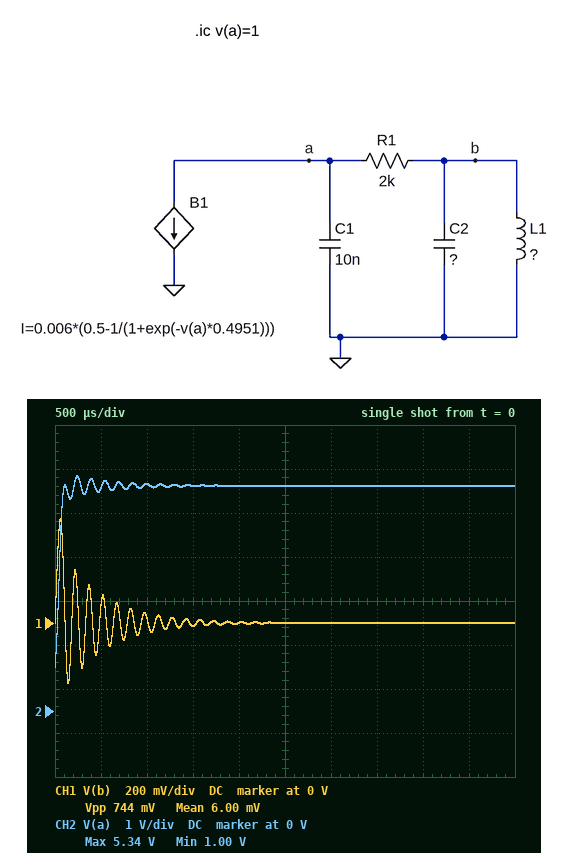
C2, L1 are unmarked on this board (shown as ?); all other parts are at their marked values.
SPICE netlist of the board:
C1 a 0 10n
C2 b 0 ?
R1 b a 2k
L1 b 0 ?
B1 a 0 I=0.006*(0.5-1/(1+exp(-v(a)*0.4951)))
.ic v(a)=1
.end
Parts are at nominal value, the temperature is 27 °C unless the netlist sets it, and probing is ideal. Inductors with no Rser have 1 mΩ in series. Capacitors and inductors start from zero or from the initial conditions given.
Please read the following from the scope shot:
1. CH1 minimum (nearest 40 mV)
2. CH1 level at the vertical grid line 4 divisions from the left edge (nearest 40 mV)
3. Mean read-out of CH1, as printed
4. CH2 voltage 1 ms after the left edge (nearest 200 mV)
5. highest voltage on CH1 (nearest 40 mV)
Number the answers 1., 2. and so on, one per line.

1. -280 mV
2. 0 V
3. 6.00 mV
4. 5.2 V
5. 480 mV
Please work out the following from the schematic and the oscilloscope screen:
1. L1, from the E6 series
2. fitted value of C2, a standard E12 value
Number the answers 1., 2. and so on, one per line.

1. 10 mH
2. 47 nF
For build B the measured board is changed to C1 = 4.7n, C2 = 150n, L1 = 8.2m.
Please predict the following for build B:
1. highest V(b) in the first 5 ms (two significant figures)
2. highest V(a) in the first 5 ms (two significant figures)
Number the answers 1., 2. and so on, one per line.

1. 1.5 V
2. 7.0 V
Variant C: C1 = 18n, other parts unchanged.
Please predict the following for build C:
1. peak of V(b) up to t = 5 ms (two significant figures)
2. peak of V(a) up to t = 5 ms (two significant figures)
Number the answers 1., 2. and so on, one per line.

1. 290 mV
2. 5.1 V
